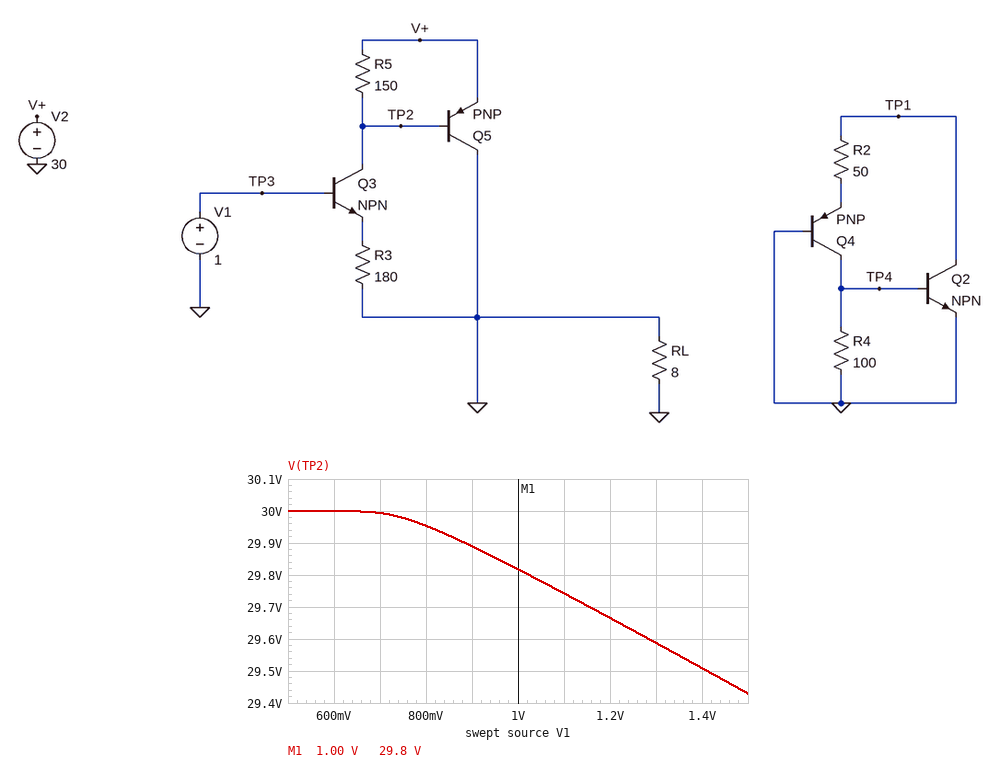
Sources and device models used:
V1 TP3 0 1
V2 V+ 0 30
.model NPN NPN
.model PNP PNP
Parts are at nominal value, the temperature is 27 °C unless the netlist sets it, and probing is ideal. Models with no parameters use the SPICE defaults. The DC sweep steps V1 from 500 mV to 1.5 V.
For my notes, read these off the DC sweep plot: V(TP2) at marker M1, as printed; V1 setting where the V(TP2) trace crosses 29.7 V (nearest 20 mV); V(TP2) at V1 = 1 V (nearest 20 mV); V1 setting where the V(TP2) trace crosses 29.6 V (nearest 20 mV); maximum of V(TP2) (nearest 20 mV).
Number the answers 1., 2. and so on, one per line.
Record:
1. 29.8 V
2. 1.16 V
3. 29.82 V
4. 1.28 V
5. 30.00 V
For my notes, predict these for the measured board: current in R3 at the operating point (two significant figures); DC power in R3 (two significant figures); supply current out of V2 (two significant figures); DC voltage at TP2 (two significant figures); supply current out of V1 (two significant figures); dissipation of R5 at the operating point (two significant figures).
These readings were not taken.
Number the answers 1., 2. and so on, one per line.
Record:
1. 1.2 mA
2. 270 µW
3. 1.2 mA
4. 30 V
5. 12 µA
6. 220 µW
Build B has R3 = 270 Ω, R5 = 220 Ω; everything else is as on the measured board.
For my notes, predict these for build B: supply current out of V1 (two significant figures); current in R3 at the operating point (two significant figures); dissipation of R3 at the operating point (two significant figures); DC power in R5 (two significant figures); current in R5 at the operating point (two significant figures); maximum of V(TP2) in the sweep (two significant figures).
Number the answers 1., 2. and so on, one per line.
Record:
1. 8.4 µA
2. 850 µA
3. 200 µW
4. 160 µW
5. 840 µA
6. 30 V
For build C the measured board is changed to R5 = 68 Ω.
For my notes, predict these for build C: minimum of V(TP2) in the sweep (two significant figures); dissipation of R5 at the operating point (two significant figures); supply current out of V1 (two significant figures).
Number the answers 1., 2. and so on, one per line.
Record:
1. 30 V
2. 100 µW
3. 12 µA
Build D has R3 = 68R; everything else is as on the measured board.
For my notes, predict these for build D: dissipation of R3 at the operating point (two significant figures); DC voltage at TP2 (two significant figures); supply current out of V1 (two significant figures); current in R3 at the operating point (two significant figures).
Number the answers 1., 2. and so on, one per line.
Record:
1. 580 µW
2. 30 V
3. 29 µA
4. 2.9 mA
